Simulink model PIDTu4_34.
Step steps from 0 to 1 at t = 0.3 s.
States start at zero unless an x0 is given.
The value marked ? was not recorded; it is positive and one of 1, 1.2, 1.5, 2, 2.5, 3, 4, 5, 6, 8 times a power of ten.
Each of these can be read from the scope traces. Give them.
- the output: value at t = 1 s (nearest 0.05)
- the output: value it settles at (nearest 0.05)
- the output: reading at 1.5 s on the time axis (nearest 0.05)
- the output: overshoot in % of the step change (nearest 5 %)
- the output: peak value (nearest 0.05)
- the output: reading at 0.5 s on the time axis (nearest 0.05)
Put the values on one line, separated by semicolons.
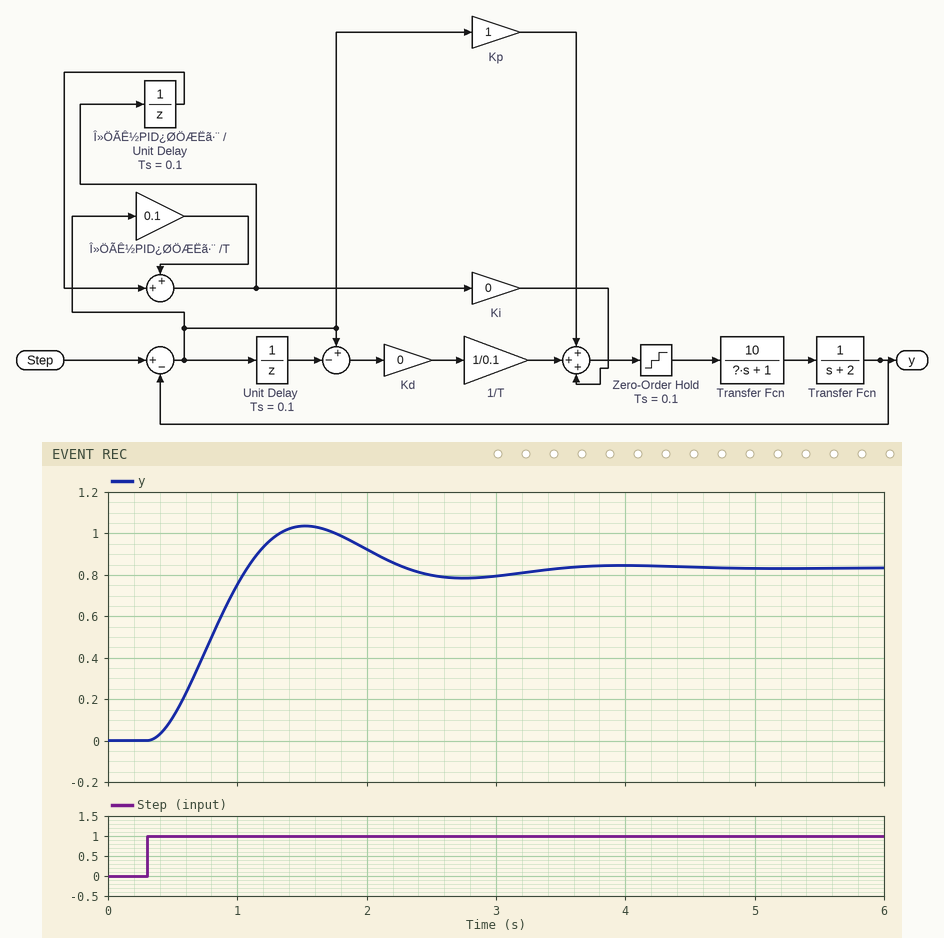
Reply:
0.75; 0.85; 1.05; 25 %; 1.05; 0.10
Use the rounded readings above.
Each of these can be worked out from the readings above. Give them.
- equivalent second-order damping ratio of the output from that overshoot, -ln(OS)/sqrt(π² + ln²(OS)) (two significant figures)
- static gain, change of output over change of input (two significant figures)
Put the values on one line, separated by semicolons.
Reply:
0.40; 0.85
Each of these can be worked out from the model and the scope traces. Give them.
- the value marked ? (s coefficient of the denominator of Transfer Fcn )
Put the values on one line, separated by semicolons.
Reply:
1.5
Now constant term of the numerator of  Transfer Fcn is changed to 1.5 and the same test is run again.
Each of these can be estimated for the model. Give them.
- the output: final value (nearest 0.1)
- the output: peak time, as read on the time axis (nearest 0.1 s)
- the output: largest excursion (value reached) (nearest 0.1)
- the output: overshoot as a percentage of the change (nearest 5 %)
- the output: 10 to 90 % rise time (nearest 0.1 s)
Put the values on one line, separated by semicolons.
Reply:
0.9; 1.3 s; 1.2; 35 %; 0.4 s
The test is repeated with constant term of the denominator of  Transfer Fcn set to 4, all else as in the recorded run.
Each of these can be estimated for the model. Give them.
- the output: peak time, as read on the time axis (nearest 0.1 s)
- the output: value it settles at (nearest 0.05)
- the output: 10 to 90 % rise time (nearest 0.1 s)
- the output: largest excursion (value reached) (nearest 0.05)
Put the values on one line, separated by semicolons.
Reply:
1.8 s; 0.70; 0.7 s; 0.75
